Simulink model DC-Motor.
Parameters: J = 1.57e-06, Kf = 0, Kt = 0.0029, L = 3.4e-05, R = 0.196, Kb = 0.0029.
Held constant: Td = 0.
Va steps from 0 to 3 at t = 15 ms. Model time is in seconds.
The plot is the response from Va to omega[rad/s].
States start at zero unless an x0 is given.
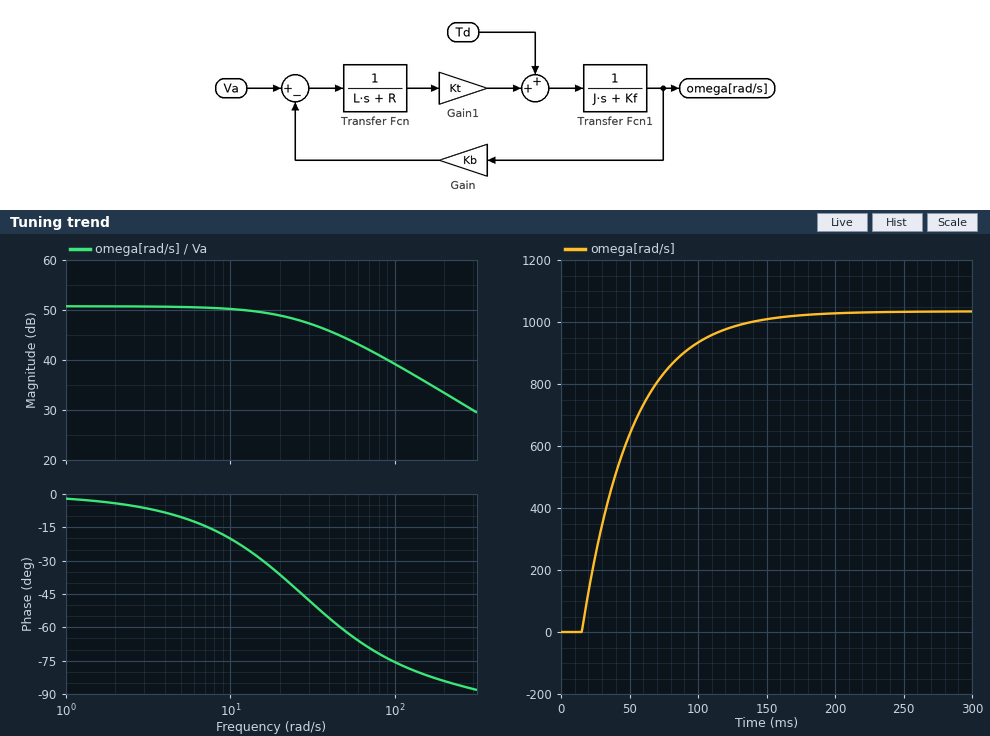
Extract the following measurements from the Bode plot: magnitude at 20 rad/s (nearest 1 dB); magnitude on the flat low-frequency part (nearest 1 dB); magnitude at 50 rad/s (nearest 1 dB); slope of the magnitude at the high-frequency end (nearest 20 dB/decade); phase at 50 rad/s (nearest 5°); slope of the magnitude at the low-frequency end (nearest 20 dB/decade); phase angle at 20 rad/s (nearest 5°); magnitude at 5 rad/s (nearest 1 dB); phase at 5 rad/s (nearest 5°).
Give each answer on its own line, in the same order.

49 dB
51 dB
44 dB
-20 dB/decade
-60°
0 dB/decade
-35°
51 dB
-10°
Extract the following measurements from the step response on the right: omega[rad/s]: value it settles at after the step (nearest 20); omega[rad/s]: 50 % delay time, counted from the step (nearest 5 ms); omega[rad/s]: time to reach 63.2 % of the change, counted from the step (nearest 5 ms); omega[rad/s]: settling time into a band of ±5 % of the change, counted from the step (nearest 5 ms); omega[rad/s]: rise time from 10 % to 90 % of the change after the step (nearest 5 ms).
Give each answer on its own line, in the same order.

1040
25 ms
35 ms
110 ms
80 ms
